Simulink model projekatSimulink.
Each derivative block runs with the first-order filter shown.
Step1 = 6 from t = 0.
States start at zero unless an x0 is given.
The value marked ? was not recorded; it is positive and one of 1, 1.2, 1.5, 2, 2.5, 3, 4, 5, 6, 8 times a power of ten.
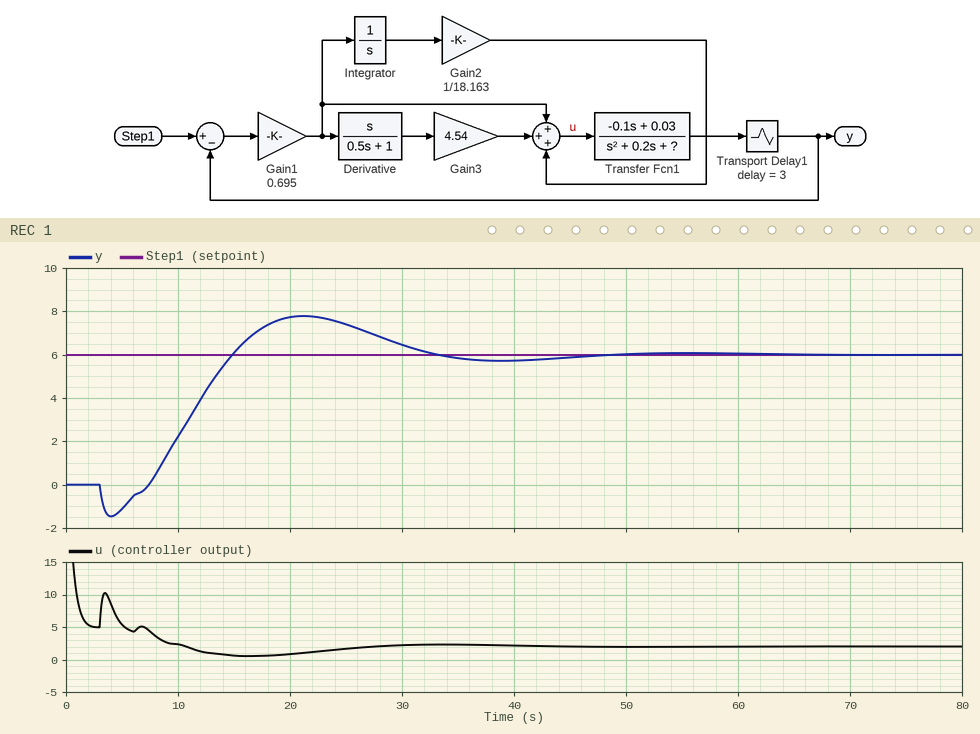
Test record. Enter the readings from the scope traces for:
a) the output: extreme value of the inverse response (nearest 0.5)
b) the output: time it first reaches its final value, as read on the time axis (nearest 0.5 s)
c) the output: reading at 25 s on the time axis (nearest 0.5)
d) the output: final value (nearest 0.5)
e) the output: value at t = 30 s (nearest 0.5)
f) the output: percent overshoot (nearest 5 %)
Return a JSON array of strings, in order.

["-1.5", "15.0 s", "7.5", "6.0", "6.5", "30 %"]
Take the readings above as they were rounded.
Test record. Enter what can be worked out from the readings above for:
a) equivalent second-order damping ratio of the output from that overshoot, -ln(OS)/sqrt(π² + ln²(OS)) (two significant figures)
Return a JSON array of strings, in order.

["0.36"]
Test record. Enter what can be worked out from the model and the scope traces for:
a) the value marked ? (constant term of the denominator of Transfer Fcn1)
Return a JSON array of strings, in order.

["0.01"]
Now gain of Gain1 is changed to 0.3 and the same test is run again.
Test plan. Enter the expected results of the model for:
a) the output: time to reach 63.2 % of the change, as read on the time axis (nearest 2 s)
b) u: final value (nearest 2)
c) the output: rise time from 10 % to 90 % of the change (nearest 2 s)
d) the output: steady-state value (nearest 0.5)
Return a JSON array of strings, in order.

["22 s", "2", "26 s", "6.0"]
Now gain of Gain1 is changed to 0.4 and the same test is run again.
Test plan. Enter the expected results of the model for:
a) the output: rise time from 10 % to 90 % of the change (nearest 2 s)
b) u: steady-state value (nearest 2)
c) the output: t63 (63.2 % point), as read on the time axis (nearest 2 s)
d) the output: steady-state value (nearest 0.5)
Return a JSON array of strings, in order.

["16 s", "2", "16 s", "6.0"]
